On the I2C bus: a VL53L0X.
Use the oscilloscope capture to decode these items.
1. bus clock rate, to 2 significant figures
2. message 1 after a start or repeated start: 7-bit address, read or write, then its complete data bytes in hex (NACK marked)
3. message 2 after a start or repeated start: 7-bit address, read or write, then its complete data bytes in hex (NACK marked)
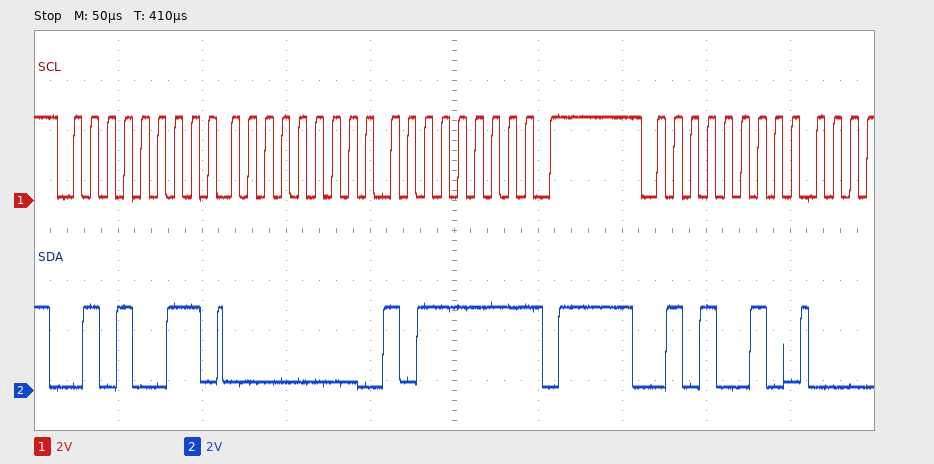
100 kHz
0x29 read: 00 BF NACK
0x29 write
